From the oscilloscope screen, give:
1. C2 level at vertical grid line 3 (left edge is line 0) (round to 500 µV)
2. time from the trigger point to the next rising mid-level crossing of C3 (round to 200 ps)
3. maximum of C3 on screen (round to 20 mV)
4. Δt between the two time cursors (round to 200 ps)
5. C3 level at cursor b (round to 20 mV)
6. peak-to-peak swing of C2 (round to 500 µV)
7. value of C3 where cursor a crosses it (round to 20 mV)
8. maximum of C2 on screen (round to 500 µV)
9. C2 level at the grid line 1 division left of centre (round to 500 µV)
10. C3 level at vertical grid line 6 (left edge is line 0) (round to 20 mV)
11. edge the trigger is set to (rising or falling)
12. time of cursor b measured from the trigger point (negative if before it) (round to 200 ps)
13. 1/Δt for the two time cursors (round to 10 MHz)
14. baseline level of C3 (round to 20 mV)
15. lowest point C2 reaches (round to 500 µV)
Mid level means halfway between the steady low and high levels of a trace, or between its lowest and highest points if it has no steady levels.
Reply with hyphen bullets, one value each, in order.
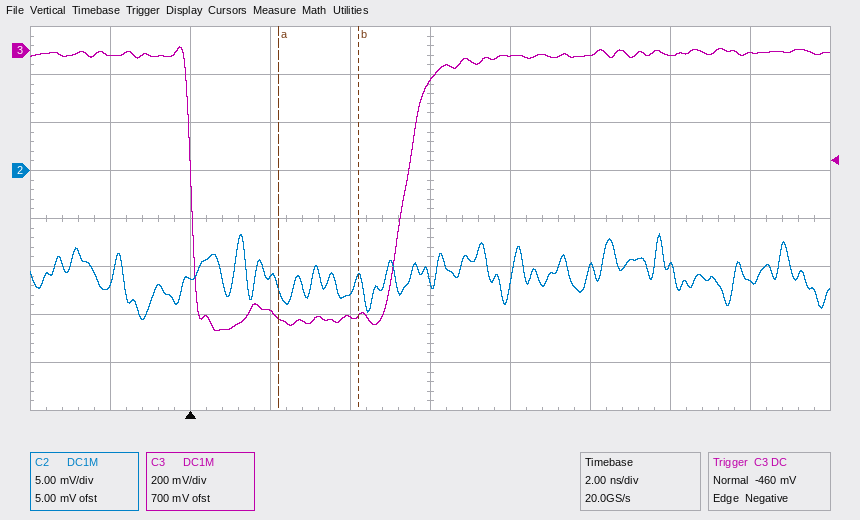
- -11.0 mV
- 5.4 ns
- 20 mV
- 2.0 ns
- -1.10 V
- 9.0 mV
- -1.12 V
- -6.5 mV
- -12.5 mV
- -20 mV
- falling
- +4.2 ns
- 500 MHz
- -20 mV
- -15.5 mV
